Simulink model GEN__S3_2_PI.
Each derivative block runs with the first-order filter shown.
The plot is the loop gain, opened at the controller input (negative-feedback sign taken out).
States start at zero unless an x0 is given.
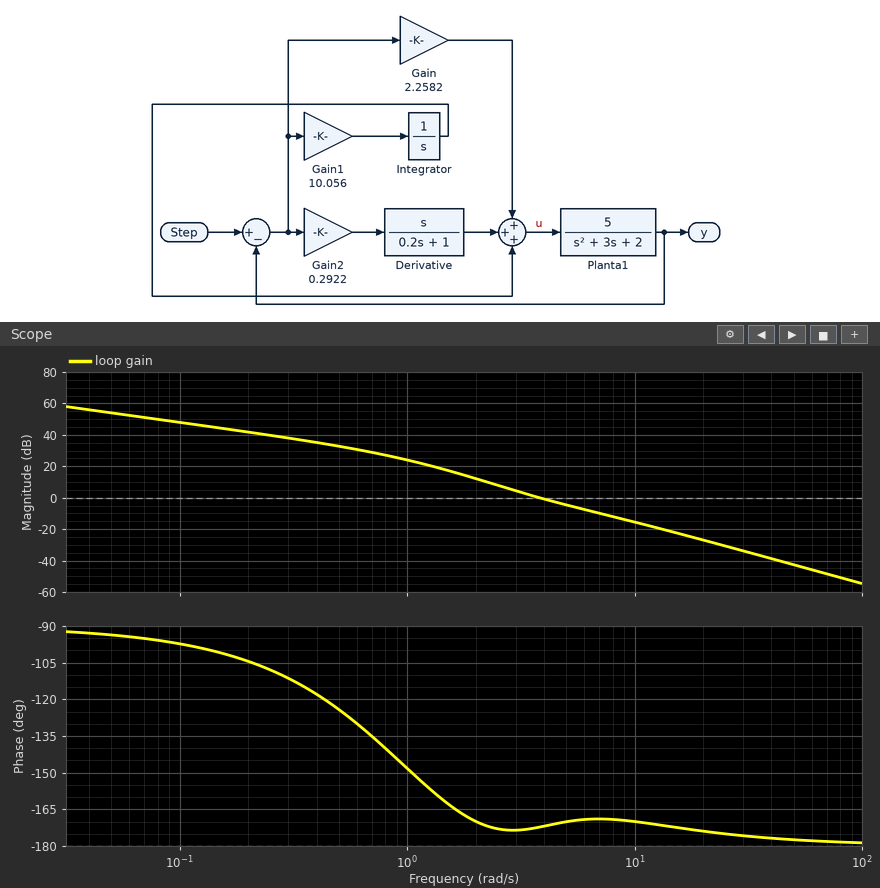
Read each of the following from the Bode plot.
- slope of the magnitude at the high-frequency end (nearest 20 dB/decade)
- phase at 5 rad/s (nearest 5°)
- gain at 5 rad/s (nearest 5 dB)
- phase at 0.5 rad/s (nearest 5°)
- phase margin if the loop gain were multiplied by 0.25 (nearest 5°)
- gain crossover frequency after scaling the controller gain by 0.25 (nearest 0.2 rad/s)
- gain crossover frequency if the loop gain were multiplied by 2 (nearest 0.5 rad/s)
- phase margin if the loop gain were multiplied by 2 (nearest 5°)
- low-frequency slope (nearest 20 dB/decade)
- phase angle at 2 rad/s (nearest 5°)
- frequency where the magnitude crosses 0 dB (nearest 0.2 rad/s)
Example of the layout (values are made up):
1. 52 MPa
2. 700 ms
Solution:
1. -40 dB/decade
2. -170°
3. -5 dB
4. -125°
5. 10°
6. 2.0 rad/s
7. 5.5 rad/s
8. 10°
9. -20 dB/decade
10. -170°
11. 3.8 rad/s
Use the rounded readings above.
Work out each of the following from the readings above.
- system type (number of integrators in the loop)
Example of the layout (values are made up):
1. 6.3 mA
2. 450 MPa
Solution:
1. 1
